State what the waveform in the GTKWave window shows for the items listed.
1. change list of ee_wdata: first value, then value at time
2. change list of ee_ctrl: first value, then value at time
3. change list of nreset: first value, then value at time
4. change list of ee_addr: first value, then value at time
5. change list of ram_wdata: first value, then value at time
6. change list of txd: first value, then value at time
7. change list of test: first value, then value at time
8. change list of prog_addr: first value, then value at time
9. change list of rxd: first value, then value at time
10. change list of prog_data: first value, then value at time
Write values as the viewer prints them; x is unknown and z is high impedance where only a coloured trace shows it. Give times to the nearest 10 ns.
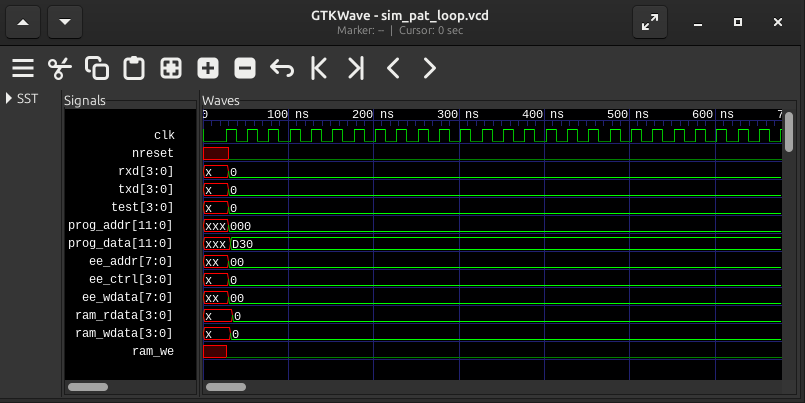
xx, 00 at 30 ns
x, 0 at 30 ns
x, 0 at 30 ns
xx, 00 at 30 ns
x, 0 at 30 ns
x, 0 at 30 ns
x, 0 at 30 ns
xxx, 000 at 30 ns
x, 0 at 30 ns
xxx, D30 at 30 ns
